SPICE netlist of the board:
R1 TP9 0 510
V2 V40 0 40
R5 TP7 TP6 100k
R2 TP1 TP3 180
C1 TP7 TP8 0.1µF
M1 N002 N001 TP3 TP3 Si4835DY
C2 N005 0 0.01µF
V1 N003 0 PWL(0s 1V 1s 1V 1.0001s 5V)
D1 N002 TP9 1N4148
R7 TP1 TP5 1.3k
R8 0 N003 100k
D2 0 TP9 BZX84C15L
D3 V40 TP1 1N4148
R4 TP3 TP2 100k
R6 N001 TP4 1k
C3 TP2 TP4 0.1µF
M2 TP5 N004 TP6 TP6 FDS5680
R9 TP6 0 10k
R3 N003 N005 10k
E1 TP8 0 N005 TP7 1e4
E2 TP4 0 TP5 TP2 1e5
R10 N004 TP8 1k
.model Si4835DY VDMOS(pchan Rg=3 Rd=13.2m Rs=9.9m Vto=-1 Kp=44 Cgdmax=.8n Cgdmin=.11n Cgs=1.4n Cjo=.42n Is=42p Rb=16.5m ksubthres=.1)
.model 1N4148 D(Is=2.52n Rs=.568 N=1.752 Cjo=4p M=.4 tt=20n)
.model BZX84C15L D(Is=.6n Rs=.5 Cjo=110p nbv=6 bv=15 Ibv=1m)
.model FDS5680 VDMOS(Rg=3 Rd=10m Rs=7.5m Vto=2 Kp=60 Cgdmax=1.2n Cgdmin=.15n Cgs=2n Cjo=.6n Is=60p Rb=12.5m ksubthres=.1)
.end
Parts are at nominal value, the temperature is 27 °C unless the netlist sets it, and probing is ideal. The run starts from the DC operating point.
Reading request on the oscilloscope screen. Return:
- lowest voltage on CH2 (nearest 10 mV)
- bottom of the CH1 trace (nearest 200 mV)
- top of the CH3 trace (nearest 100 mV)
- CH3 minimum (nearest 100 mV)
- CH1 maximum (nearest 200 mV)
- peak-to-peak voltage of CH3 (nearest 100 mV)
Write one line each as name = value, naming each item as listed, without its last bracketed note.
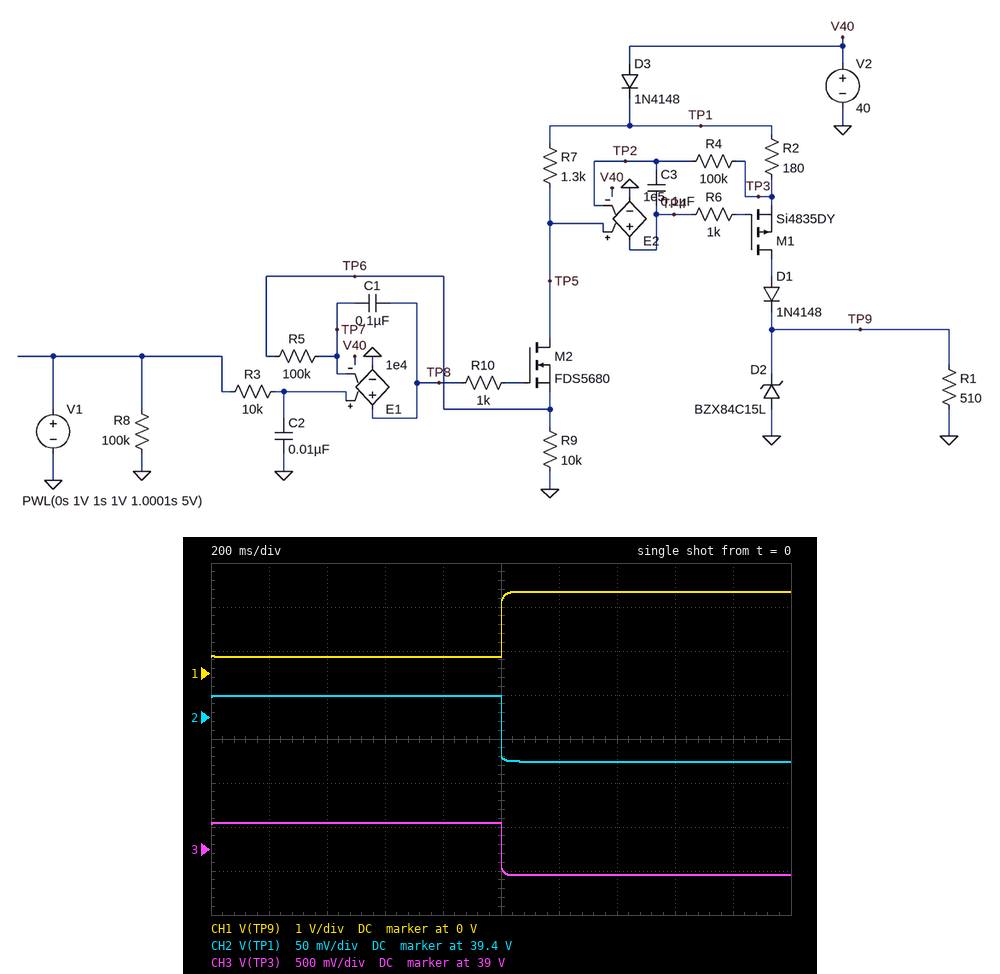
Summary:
lowest voltage on CH2 = 39.35 V
bottom of the CH1 trace = 400 mV
top of the CH3 trace = 39.3 V
CH3 minimum = 38.7 V
CH1 maximum = 1.8 V
peak-to-peak voltage of CH3 = 600 mV
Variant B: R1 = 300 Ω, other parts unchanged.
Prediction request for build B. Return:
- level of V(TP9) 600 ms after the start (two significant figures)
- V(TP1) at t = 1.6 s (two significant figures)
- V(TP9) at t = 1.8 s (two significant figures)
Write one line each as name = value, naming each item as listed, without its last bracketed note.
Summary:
level of V(TP9) 600 ms after the start = 220 mV
V(TP1) at t = 1.6 s = 39 V
V(TP9) at t = 1.8 s = 1.1 V
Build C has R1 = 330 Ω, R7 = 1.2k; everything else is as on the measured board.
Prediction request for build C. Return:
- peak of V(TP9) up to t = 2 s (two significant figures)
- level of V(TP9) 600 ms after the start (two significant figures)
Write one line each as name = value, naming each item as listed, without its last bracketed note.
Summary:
peak of V(TP9) up to t = 2 s = 1.1 V
level of V(TP9) 600 ms after the start = 220 mV
